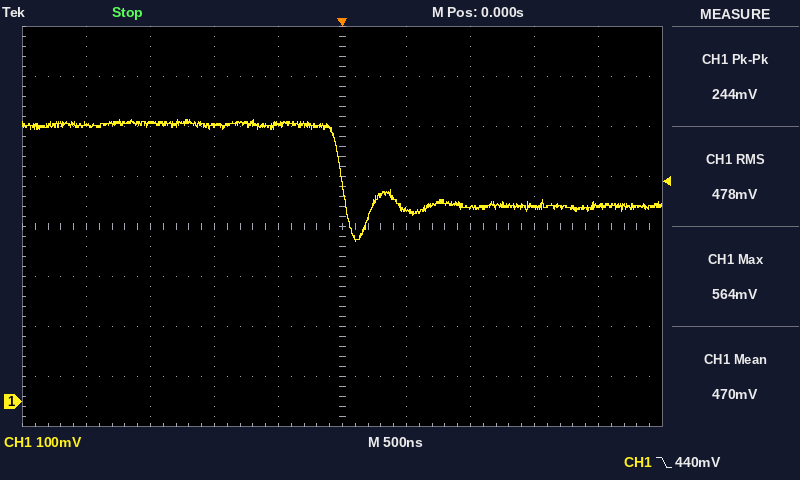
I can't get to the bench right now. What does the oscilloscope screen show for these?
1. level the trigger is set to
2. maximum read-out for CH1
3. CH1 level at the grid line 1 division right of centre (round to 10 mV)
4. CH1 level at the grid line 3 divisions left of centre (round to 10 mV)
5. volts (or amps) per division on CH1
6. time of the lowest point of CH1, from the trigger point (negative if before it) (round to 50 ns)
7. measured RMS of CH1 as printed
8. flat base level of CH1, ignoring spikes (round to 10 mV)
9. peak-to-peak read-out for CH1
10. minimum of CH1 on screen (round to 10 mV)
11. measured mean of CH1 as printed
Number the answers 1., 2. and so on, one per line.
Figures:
1. 440 mV
2. 564 mV
3. 380 mV
4. 560 mV
5. 100 mV
6. +100 ns
7. 478 mV
8. 390 mV
9. 244 mV
10. 320 mV
11. 470 mV
